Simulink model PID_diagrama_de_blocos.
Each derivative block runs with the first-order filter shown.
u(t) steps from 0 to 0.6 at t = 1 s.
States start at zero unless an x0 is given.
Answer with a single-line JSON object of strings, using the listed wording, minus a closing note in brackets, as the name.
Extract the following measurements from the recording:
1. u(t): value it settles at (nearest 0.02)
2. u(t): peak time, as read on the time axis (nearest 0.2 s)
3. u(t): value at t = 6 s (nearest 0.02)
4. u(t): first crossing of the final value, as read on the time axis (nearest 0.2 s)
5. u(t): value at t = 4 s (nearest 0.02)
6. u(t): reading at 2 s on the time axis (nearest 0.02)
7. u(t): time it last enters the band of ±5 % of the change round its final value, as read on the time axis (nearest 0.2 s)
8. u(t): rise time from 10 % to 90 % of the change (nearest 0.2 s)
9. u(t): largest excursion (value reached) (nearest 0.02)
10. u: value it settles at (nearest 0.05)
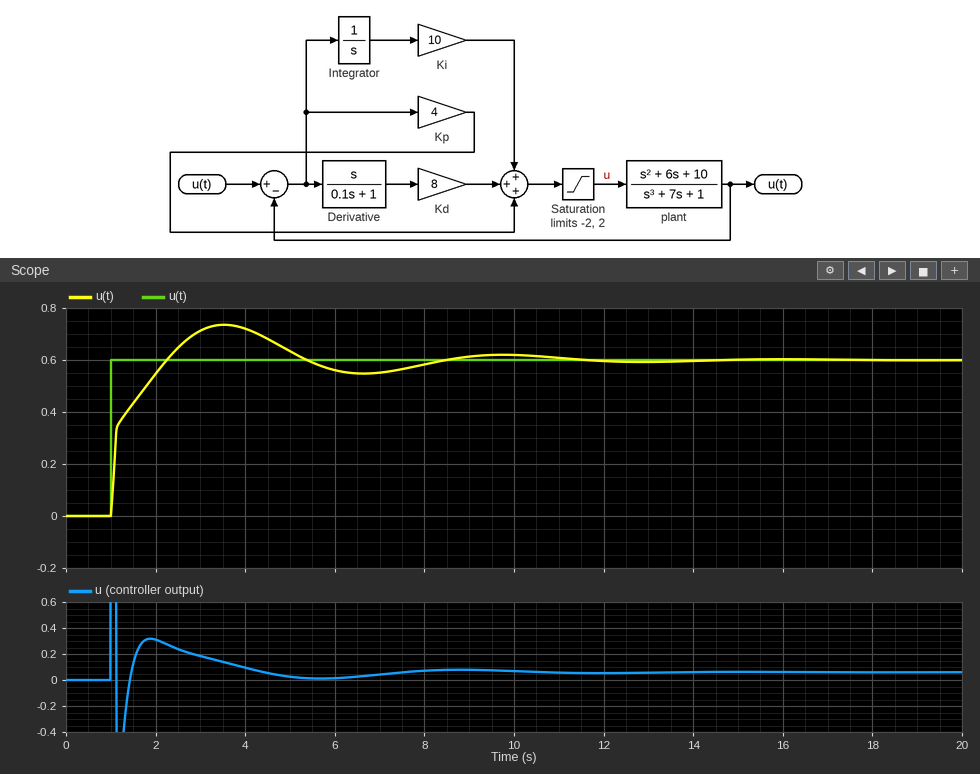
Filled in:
{"u(t): value it settles at": "0.60", "u(t): peak time, as read on the time axis": "3.6 s", "u(t): value at t = 6 s": "0.56", "u(t): first crossing of the final value, as read on the time axis": "2.2 s", "u(t): value at t = 4 s": "0.72", "u(t): reading at 2 s on the time axis": "0.54", "u(t): time it last enters the band of ±5 % of the change round its final value, as read on the time axis": "7.6 s", "u(t): rise time from 10 % to 90 % of the change": "1.0 s", "u(t): largest excursion (value reached)": "0.74", "u: value it settles at": "0.05"}
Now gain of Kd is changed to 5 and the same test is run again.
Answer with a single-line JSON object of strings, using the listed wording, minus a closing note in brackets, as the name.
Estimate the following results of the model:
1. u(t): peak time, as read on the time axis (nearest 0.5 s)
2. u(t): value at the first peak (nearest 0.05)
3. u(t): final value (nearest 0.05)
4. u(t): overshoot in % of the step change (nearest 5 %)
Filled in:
{"u(t): peak time, as read on the time axis": "3.0 s", "u(t): value at the first peak": "0.70", "u(t): final value": "0.60", "u(t): overshoot in % of the step change": "20 %"}
